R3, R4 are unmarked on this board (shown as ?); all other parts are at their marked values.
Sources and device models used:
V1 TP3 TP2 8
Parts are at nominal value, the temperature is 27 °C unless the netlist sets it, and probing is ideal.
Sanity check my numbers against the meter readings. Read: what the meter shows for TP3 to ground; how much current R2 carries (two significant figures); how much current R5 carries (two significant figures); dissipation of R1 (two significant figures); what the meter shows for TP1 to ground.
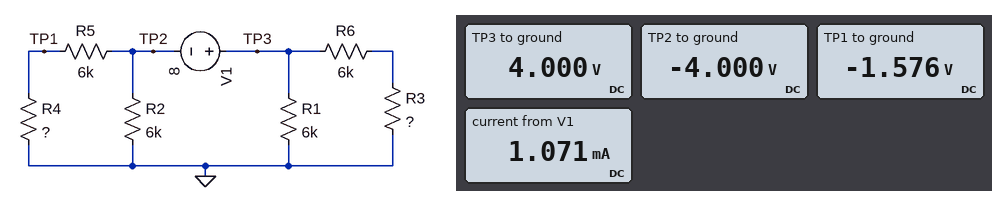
4.000 V
670 µA
400 µA
2.7 mW
-1.576 V
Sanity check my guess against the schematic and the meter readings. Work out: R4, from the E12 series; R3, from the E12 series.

3.9 kΩ
3.9 kΩ
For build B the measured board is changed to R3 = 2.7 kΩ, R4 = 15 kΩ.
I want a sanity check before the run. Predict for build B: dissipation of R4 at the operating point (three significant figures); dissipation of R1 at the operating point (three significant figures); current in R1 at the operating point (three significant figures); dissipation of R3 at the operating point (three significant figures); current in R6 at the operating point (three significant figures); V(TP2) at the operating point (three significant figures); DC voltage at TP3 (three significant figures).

702 µW
1.99 mW
576 µA
426 µW
397 µA
-4.54 V
3.46 V
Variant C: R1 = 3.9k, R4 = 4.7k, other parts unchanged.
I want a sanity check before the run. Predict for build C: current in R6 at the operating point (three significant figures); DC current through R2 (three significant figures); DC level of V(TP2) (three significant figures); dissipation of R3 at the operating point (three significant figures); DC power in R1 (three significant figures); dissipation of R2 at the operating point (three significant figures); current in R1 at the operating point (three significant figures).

340 µA
772 µA
-4.63 V
452 µW
2.91 mW
3.57 mW
864 µA
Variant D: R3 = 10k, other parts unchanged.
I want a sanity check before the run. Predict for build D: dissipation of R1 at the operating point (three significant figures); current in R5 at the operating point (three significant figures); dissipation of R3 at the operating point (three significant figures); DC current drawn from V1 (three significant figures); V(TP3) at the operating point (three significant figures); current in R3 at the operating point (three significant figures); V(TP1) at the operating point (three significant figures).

3.10 mW
373 µA
726 µW
988 µA
4.31 V
269 µA
-1.45 V
